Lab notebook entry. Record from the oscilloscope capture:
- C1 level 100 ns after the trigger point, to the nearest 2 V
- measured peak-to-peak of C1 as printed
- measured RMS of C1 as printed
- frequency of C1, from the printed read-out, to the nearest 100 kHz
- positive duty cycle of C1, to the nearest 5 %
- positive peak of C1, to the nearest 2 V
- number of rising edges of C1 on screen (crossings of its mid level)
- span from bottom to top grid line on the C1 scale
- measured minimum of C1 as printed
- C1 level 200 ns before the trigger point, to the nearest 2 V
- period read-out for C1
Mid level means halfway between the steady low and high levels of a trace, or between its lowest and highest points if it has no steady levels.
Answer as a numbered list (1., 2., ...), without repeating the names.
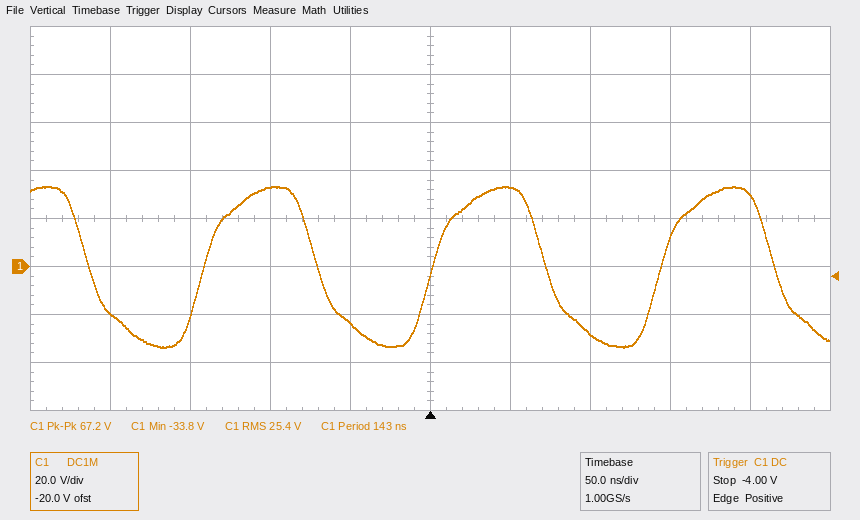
1. -28 V
2. 67.2 V
3. 25.4 V
4. 7.0 MHz
5. 50 %
6. 34 V
7. 3
8. 160 V
9. -33.8 V
10. -20 V
11. 143 ns
